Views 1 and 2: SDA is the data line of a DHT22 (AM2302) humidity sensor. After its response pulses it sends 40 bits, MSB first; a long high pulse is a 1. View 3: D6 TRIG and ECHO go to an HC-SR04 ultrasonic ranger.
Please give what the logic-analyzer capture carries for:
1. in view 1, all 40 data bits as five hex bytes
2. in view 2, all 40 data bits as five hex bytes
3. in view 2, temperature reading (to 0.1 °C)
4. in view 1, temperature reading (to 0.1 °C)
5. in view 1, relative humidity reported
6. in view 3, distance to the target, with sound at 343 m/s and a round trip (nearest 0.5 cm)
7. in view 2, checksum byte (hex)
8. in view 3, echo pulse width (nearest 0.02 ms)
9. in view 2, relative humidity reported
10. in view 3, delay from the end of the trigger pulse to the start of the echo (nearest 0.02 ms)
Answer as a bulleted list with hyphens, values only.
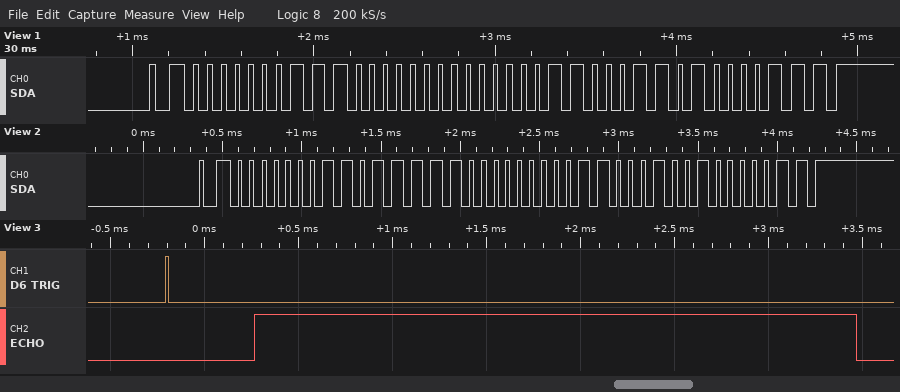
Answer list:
- 01 C0 00 C6 87
- 01 BE 00 C4 83
- 19.6 °C
- 19.8 °C
- 44.8 %
- 55 cm
- 0x83
- 3.20 ms
- 44.6 %
- 0.46 ms
